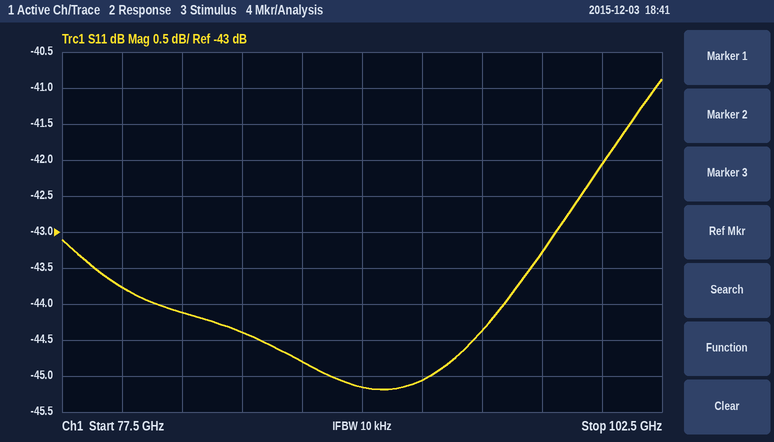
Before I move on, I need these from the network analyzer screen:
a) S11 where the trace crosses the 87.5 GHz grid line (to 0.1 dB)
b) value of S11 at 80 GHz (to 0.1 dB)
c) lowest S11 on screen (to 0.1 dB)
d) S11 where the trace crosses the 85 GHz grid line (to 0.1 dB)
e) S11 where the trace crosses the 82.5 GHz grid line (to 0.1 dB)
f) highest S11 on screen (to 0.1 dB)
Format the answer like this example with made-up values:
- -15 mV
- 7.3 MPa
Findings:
- -44.8 dB
- -43.8 dB
- -45.2 dB
- -44.4 dB
- -44.1 dB
- -40.9 dB
